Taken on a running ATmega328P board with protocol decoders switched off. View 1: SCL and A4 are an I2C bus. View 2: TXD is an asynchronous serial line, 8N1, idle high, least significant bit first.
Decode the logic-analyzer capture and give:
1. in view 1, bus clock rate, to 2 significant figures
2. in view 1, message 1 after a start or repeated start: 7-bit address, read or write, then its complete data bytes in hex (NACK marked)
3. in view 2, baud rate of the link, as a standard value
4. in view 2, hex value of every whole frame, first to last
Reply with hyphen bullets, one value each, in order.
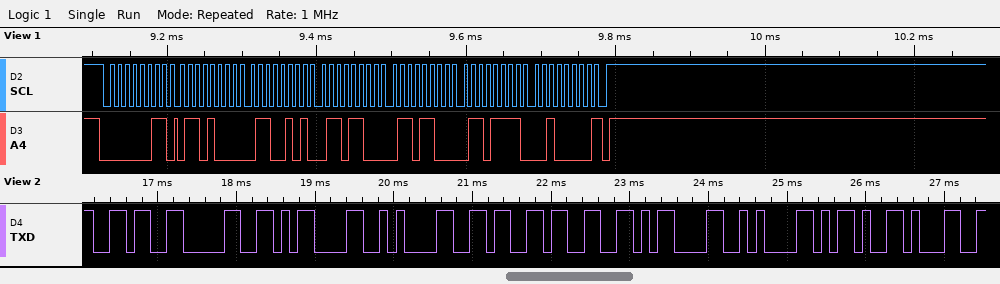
- 100 kHz
- 0x01 read: 68 65 6C 6C 6F 20 NACK
- 9600 baud
- 36 30 0D 0A 36 33 0D 0A 2D 31
